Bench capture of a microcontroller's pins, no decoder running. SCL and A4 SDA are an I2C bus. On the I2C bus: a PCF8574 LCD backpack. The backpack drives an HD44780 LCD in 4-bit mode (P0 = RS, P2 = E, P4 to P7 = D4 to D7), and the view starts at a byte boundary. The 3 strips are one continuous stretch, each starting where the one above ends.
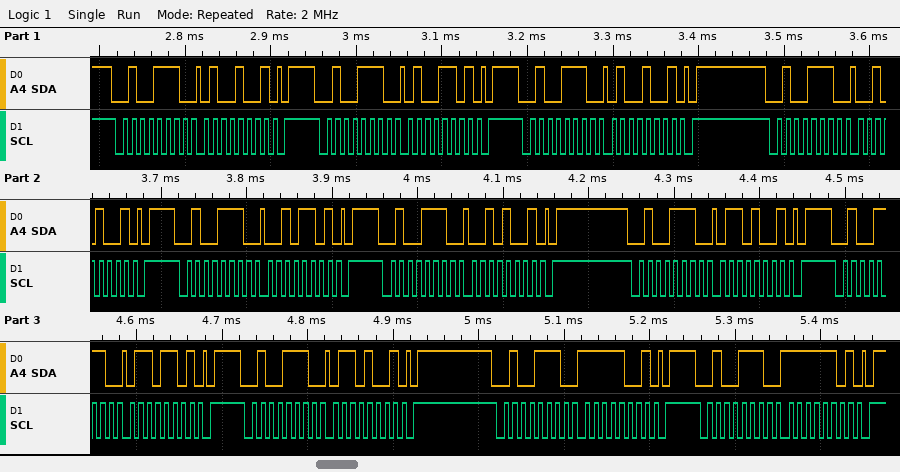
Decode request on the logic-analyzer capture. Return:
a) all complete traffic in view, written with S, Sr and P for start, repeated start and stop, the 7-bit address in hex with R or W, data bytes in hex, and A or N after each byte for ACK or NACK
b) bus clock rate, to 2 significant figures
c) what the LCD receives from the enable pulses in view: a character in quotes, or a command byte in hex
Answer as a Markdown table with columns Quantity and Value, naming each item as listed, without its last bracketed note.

| Quantity | Value |
|---|---|
| all complete traffic in view, written with S, Sr and P for start, repeated start and stop, the 7-bit address in hex with R or W, data bytes in hex, and A or N after each byte for ACK or NACK | S 27W A 49 A P S 27W A 4D A P S 27W A 49 A P S 27W A 29 A P S 27W A 2D A P S 27W A 29 A P S 27W A 69 A P S 27W A 6D A P S 27W A 69 A P S 27W A F9 A P S 27W A FD A P |
| bus clock rate, to 2 significant figures | 100 kHz |
| what the LCD receives from the enable pulses in view: a character in quotes, or a command byte in hex | 'B' |
